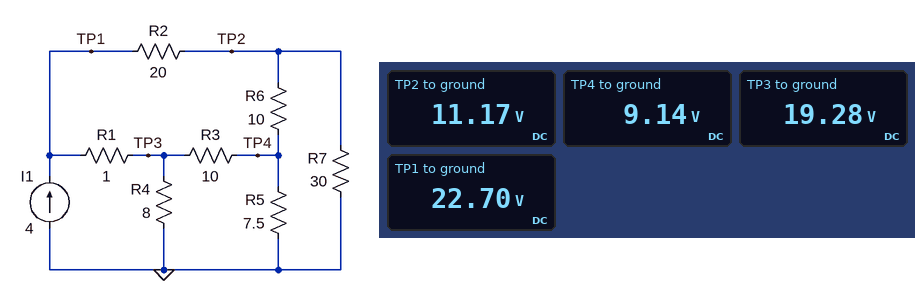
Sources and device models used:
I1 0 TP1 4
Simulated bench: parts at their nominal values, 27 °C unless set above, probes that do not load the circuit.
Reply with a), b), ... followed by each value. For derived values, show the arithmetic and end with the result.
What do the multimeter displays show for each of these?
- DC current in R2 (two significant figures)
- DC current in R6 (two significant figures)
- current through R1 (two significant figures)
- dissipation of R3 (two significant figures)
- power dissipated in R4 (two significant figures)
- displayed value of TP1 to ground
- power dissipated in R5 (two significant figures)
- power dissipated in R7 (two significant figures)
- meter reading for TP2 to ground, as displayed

a) (22.7 V - 11.17 V) / 20 Ω = 580 mA
b) (11.17 V - 9.14 V) / 10 Ω = 200 mA
c) (22.7 V - 19.28 V) / 1 Ω = 3.4 A
d) (19.28 V - 9.14 V)^2 / 10 Ω = 10 W
e) (19.28 V)^2 / 8 Ω = 46 W
f) 22.70 V
g) (9.14 V)^2 / 7.5 Ω = 11 W
h) (11.17 V)^2 / 30 Ω = 4.2 W
i) 11.17 V
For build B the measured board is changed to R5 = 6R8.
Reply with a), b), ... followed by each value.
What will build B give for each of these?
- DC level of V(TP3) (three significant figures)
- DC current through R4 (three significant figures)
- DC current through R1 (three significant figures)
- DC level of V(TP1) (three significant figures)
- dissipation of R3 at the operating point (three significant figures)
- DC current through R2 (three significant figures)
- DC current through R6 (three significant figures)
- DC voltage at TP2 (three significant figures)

a) 19.0 V
b) 2.38 A
c) 3.42 A
d) 22.4 V
e) 10.9 W
f) 581 mA
g) 221 mA
h) 10.8 V
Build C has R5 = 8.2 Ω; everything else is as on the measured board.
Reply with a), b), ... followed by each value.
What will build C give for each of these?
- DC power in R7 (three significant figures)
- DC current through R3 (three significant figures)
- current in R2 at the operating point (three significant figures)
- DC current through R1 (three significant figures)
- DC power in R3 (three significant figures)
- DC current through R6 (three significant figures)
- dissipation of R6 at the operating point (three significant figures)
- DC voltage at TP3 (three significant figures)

a) 4.42 W
b) 988 mA
c) 572 mA
d) 3.43 A
e) 9.76 W
f) 188 mA
g) 352 mW
h) 19.5 V
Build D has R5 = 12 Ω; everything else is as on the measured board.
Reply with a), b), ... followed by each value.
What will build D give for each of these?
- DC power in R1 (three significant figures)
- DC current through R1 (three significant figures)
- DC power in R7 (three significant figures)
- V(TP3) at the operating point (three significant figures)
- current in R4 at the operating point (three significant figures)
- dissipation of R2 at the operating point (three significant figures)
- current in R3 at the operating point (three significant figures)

a) 11.9 W
b) 3.45 A
c) 5.67 W
d) 20.6 V
e) 2.58 A
f) 6.07 W
g) 873 mA
